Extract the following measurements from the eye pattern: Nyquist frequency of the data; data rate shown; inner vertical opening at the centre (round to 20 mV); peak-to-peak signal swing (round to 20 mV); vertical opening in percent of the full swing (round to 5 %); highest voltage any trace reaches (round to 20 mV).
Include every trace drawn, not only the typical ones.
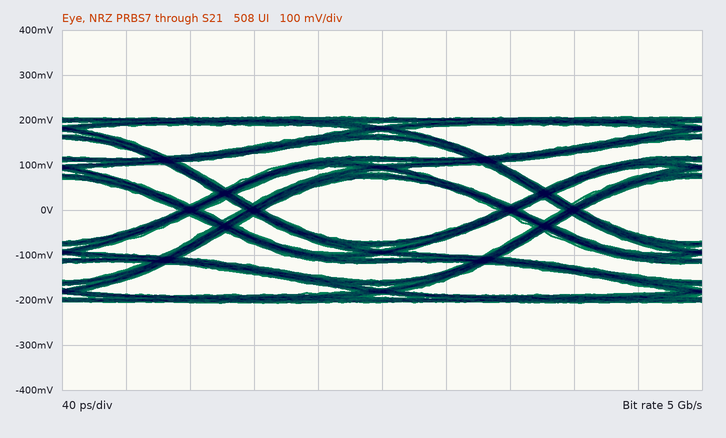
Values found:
2.5 GHz
5 Gb/s
140 mV
420 mV
35 %
200 mV
